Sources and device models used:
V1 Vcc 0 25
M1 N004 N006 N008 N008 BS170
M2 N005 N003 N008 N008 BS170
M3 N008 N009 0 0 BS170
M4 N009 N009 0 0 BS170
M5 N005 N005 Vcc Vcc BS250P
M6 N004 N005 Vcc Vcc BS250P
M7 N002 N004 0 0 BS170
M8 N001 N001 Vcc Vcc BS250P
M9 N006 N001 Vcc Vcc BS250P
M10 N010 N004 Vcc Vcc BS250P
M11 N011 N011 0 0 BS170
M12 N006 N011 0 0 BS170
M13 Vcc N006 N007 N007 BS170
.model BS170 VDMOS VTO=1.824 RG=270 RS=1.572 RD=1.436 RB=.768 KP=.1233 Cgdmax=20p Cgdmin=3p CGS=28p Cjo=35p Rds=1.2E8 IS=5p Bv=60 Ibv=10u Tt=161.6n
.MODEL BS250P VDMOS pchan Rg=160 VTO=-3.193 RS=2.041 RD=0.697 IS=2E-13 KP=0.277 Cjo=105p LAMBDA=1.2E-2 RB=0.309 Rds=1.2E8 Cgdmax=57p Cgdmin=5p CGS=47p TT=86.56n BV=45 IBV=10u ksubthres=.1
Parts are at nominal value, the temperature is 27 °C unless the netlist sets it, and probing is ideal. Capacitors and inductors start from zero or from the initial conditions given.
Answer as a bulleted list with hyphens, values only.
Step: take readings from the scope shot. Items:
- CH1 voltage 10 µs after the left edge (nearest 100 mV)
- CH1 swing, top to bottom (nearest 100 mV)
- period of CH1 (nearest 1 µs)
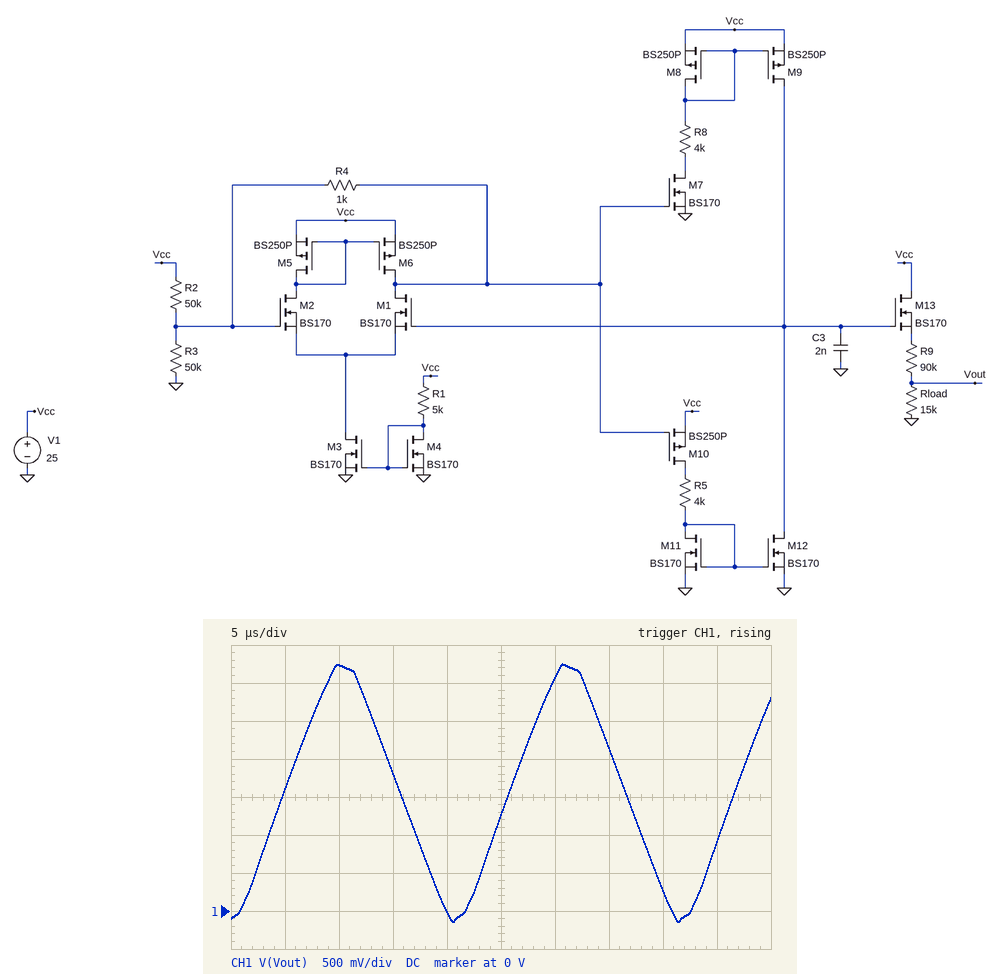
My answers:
- 3.2 V
- 3.4 V
- 21 µs
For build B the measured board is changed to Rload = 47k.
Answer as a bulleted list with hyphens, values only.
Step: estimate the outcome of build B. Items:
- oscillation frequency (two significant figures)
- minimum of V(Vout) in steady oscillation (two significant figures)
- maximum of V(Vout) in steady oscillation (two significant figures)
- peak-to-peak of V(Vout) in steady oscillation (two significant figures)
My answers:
- 48 kHz
- -330 mV
- 7.8 V
- 8.1 V
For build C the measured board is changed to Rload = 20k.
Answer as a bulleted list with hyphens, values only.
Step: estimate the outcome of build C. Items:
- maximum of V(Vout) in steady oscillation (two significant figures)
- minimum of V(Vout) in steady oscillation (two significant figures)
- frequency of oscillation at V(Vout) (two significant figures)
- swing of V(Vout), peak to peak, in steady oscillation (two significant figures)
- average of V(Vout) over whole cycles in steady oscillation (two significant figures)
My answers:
- 4.1 V
- -180 mV
- 48 kHz
- 4.3 V
- 2.0 V
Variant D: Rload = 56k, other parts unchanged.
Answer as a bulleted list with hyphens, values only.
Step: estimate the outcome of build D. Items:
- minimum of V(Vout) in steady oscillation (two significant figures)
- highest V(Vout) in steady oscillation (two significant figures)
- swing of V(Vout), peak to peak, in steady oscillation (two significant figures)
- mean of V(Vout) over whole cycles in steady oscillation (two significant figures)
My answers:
- -370 mV
- 8.7 V
- 9.1 V
- 4.3 V
